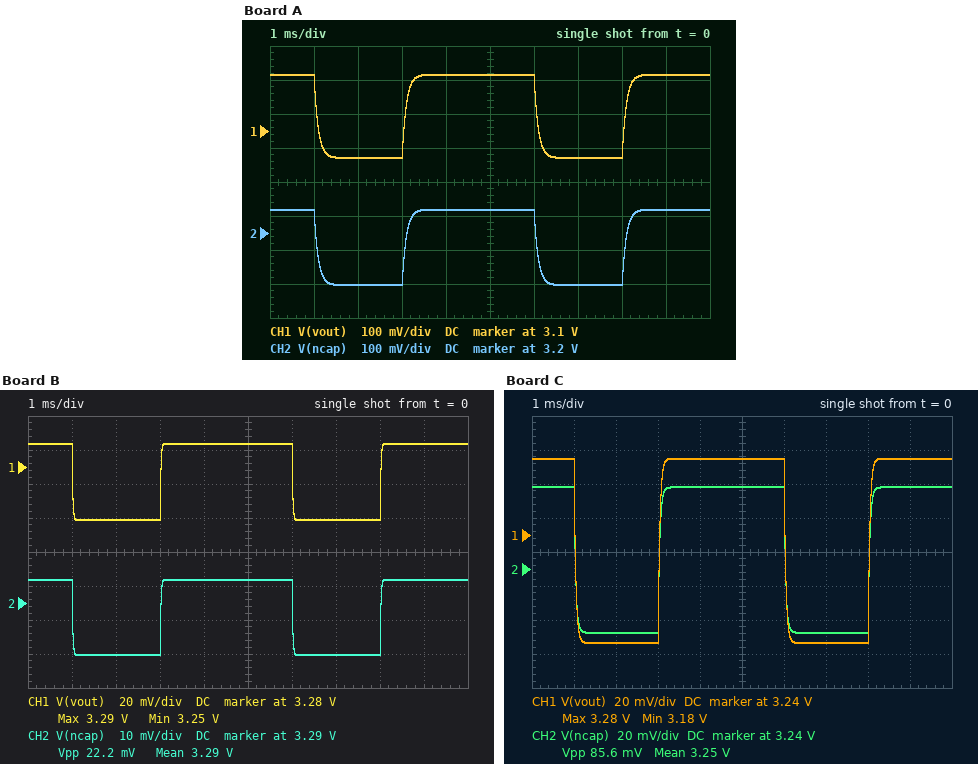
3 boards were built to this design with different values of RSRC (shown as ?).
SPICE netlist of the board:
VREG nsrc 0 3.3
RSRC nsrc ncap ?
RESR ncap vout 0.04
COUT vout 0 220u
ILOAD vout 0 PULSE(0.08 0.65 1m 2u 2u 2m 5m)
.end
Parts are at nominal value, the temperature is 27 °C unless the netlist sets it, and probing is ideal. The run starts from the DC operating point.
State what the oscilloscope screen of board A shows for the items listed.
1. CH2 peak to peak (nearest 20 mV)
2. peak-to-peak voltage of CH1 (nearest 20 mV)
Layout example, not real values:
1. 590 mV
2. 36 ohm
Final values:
1. 220 mV
2. 240 mV
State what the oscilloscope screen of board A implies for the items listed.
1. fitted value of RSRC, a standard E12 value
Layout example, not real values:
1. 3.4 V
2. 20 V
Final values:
1. 0.39 Ω
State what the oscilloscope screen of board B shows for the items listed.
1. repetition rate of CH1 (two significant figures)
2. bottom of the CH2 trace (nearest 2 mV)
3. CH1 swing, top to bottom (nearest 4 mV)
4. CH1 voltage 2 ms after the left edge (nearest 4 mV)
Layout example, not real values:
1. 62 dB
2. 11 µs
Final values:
1. 200 Hz
2. 3.274 V
3. 44 mV
4. 3.248 V
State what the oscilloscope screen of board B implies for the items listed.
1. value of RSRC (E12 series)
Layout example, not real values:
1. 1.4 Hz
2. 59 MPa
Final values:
1. 0.039 Ω
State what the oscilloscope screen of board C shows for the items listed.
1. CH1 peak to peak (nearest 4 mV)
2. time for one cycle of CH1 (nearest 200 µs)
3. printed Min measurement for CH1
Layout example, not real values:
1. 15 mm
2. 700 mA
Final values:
1. 108 mV
2. 5.0 ms
3. 3.18 V
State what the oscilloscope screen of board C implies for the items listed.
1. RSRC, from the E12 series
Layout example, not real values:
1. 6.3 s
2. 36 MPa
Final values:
1. 0.15 Ω
